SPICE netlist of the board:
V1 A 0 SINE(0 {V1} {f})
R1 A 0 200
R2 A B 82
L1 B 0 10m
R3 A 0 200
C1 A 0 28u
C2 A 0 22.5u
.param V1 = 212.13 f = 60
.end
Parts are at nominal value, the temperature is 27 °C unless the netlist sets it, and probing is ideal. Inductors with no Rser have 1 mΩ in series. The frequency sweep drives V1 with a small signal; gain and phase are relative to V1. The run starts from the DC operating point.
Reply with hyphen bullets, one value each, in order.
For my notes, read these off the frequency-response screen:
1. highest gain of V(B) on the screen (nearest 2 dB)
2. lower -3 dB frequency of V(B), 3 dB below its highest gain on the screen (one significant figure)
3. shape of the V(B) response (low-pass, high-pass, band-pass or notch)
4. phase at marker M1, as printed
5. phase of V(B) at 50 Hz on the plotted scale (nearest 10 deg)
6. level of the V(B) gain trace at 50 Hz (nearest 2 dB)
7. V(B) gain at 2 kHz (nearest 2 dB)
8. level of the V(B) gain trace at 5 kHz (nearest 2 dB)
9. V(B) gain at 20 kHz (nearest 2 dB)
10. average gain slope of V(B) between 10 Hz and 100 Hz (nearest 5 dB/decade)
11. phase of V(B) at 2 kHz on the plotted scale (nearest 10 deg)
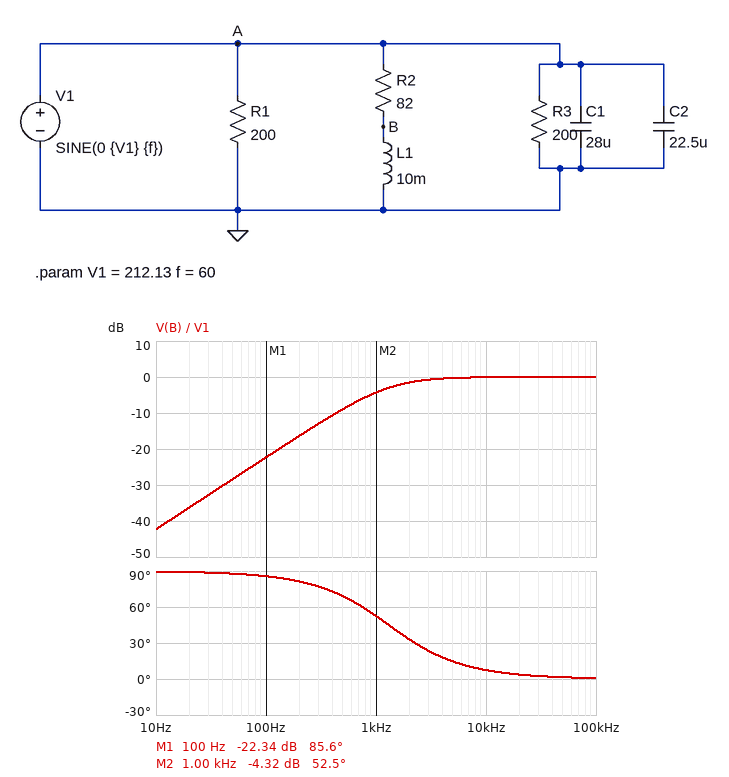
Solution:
- 0 dB
- 1 kHz
- high-pass
- 85.6 deg
- 90 deg
- -28 dB
- -2 dB
- 0 dB
- 0 dB
- 20 dB/decade
- 30 deg
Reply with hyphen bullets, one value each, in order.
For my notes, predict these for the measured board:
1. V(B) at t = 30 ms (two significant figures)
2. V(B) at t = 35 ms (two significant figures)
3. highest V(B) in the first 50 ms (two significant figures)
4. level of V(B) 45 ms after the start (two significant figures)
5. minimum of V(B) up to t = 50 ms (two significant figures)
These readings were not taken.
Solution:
- 2.6 V
- 8.1 V
- 9.7 V
- -3.4 V
- -9.7 V
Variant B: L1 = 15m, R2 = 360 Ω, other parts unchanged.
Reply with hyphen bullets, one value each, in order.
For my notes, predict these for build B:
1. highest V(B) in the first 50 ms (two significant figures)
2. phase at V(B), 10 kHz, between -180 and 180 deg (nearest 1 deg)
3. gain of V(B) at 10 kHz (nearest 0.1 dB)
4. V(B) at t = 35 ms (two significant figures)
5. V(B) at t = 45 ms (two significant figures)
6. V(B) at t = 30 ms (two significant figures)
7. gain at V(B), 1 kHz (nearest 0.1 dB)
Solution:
- 3.3 V
- 21 deg
- -0.6 dB
- 2.7 V
- -1.1 V
- 980 mV
- -11.9 dB
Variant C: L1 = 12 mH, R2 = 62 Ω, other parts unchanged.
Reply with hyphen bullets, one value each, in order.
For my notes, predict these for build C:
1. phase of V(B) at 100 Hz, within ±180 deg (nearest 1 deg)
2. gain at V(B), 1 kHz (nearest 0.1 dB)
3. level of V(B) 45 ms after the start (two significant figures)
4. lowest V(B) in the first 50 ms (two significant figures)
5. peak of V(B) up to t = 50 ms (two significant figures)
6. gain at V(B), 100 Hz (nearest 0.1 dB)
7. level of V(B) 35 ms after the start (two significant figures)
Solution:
- 83 deg
- -2.2 dB
- -5.8 V
- -15 V
- 15 V
- -18.4 dB
- 13 V
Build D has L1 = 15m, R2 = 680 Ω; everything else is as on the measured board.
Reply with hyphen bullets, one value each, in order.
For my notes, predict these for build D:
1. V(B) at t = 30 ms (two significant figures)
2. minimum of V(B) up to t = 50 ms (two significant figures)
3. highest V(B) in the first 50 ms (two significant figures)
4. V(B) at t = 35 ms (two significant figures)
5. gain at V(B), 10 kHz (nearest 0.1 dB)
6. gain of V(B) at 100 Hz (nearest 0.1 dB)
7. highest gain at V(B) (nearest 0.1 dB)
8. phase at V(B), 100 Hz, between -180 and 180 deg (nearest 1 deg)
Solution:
- 530 mV
- -1.8 V
- 1.8 V
- 1.4 V
- -1.8 dB
- -37.2 dB
- 0 dB
- 89 deg
